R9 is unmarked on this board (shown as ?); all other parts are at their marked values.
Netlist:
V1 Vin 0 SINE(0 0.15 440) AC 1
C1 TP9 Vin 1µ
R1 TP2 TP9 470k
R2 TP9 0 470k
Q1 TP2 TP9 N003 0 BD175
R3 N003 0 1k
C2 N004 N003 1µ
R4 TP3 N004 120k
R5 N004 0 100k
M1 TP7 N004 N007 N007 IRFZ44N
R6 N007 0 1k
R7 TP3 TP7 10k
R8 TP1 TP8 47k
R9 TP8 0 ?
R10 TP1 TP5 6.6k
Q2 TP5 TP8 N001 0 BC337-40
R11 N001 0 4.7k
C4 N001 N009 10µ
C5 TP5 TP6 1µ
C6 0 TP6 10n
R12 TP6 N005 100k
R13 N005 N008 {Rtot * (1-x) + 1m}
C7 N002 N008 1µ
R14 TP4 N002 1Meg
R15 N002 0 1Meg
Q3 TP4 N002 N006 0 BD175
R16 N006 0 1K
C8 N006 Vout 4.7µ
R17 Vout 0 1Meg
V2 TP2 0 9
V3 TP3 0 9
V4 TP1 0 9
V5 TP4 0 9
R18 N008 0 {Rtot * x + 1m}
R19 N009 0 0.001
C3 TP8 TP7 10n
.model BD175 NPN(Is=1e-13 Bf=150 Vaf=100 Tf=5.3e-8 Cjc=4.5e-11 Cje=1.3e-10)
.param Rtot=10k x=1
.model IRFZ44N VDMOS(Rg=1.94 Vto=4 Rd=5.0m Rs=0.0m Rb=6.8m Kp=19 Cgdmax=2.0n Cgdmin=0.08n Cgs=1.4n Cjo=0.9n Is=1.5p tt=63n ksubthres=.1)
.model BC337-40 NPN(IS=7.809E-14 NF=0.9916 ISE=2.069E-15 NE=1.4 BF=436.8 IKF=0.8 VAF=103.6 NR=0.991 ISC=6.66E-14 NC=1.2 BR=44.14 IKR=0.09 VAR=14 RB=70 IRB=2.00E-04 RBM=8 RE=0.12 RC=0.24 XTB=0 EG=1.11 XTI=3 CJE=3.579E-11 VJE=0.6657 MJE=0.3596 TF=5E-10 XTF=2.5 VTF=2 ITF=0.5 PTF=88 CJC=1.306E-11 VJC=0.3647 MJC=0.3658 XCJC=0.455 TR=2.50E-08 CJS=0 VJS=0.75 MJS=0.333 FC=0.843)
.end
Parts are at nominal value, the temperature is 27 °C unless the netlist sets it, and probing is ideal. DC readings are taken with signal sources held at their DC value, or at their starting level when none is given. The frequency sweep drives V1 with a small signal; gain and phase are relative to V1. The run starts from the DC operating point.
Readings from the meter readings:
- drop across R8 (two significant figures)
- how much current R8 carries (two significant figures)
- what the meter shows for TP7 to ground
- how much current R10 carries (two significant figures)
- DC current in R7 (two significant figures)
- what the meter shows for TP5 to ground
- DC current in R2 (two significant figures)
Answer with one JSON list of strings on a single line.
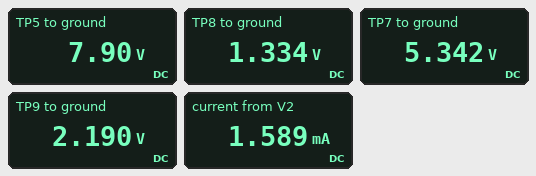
["7.7 V", "160 µA", "5.342 V", "170 µA", "370 µA", "7.90 V", "4.7 µA"]
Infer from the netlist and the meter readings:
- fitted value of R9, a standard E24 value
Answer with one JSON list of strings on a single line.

["8.2 kΩ"]
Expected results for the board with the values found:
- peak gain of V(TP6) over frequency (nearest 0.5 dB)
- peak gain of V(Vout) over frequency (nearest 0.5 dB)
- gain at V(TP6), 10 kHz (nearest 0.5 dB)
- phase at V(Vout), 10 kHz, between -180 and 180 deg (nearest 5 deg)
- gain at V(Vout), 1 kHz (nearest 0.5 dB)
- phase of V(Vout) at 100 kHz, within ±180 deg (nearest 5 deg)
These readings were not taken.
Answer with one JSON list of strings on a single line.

["39.5 dB", "17.5 dB", "30.0 dB", "-85 deg", "17.0 dB", "160 deg"]
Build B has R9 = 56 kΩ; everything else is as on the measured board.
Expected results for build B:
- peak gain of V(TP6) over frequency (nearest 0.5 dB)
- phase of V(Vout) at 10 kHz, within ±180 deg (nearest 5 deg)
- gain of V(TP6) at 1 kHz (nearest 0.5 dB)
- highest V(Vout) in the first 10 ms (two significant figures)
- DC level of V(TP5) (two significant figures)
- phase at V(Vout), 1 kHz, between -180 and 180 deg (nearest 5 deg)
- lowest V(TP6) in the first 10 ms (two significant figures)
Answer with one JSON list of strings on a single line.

["-2.5 dB", "0 deg", "-7.5 dB", "400 mV", "3.8 V", "55 deg", "-280 mV"]
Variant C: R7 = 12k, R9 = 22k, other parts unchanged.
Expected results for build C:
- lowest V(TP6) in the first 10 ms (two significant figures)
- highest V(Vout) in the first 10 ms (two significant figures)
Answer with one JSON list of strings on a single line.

["-3.5 V", "250 mV"]
